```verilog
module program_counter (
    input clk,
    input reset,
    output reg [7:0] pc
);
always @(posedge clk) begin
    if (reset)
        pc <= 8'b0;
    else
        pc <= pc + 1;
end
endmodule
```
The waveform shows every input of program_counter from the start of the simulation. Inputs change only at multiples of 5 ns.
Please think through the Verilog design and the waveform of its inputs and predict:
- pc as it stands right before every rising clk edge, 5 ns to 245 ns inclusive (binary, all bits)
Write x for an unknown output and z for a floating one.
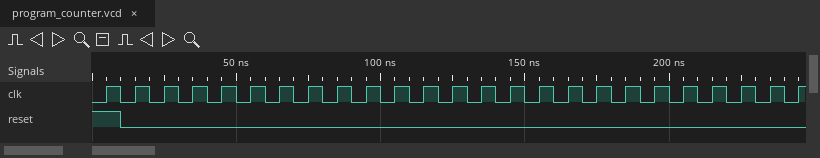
x, 00000000, 00000001, 00000010, 00000011, 00000100, 00000101, 00000110, 00000111, 00001000, 00001001, 00001010, 00001011, 00001100, 00001101, 00001110, 00001111, 00010000, 00010001, 00010010, 00010011, 00010100, 00010101, 00010110, 00010111
